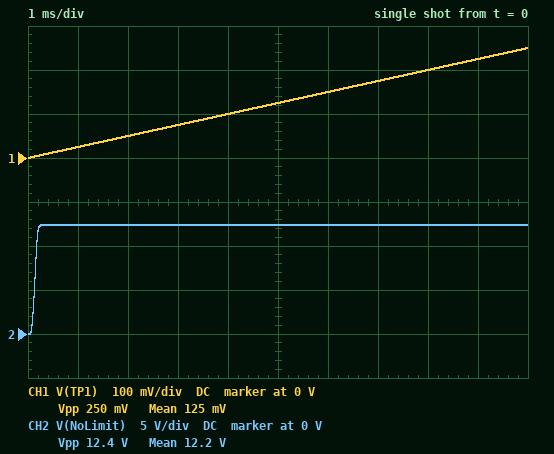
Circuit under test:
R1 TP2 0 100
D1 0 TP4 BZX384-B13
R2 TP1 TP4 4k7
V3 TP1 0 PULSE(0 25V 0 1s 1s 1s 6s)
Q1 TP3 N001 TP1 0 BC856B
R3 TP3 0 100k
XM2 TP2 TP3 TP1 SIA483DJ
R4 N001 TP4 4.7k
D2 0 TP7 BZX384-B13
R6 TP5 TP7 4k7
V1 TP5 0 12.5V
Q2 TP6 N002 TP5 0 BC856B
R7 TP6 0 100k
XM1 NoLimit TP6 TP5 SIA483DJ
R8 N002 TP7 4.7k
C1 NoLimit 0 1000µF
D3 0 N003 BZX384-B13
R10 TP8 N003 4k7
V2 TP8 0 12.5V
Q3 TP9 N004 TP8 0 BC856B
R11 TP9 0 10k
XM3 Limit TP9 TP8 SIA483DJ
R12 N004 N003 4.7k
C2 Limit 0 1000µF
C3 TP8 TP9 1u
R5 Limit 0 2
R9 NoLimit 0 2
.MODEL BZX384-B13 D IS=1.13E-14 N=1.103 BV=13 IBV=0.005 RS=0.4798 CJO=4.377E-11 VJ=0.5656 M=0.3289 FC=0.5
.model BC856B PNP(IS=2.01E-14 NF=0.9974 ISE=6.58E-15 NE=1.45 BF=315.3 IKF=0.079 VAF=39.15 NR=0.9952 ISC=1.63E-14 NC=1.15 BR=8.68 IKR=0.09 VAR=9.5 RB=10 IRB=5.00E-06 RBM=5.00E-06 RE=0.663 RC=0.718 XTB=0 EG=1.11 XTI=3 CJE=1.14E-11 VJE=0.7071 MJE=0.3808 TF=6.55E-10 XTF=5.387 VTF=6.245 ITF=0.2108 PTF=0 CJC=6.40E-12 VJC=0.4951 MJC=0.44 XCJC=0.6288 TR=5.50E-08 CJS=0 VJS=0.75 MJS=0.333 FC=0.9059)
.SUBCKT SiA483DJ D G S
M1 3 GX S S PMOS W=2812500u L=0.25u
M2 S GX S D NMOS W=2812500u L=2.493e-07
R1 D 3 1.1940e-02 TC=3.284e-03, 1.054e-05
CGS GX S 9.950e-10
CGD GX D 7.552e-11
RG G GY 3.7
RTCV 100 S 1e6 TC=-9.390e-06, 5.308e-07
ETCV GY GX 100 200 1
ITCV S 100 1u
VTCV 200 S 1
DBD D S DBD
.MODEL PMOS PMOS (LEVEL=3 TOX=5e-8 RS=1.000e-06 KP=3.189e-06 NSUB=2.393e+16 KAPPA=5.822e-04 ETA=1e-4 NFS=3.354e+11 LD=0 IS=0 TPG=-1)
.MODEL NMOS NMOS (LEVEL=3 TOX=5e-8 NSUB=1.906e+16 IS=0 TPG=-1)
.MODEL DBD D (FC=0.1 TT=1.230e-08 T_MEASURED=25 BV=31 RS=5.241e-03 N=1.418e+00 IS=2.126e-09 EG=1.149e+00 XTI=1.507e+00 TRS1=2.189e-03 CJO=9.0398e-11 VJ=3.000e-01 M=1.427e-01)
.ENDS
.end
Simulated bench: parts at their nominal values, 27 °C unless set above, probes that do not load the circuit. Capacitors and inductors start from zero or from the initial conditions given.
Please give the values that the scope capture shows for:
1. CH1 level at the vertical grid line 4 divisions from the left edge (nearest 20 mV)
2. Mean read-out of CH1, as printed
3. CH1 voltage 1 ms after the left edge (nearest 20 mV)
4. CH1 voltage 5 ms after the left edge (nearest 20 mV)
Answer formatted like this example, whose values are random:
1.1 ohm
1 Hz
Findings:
100 mV
125 mV
20 mV
120 mV
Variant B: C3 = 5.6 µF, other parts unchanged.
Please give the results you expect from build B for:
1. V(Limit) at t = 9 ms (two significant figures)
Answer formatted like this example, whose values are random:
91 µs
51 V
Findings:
1.7 mV
